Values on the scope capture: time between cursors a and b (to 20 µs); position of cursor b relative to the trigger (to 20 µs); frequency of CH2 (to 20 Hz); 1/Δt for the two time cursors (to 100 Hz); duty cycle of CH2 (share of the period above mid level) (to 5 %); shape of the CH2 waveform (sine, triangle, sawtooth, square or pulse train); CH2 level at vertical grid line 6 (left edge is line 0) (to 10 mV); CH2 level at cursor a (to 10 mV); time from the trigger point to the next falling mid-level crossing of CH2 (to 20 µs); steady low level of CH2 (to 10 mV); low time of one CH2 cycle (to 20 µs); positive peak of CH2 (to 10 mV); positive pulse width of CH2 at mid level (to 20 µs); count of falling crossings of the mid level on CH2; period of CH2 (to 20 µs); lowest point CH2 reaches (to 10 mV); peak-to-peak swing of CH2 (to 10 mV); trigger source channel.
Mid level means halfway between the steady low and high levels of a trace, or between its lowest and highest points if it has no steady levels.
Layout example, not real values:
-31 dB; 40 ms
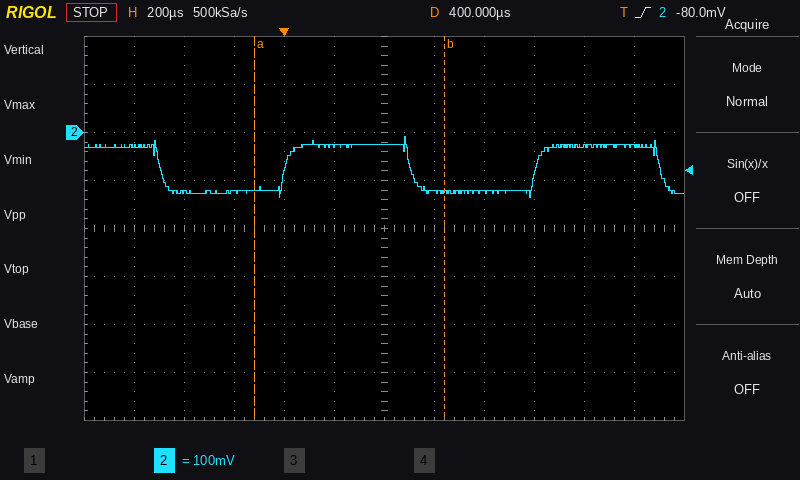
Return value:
760 µs; +640 µs; 1.00 kHz; 1.3 kHz; 50 %; square; -20 mV; -120 mV; 500 µs; -120 mV; 500 µs; -10 mV; 500 µs; 3; 1.00 ms; -140 mV; 130 mV; CH2
